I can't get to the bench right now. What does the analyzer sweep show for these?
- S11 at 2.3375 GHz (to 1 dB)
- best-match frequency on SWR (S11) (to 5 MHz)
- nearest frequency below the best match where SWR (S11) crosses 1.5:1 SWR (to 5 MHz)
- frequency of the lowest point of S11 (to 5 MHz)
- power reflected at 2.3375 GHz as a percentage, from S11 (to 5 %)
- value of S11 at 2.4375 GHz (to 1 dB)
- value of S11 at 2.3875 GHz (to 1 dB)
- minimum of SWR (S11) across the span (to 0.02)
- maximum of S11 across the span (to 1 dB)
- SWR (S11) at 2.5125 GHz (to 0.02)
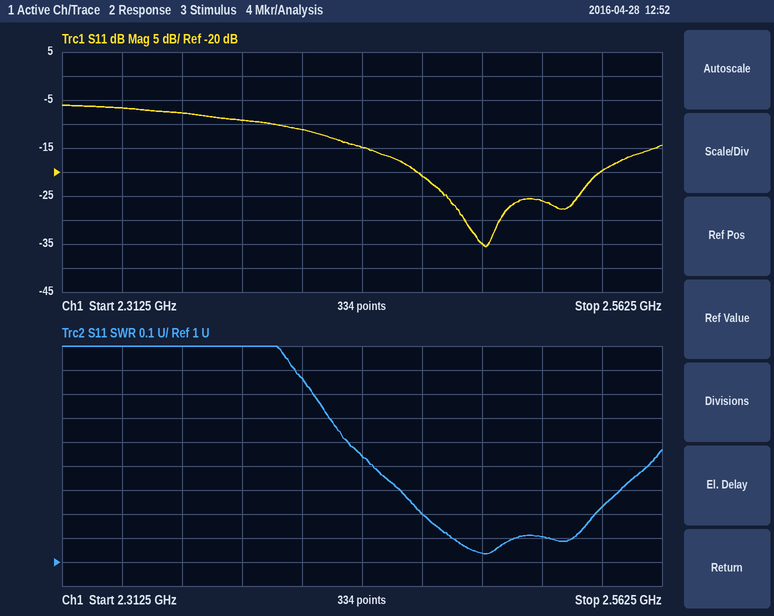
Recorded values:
-7 dB
2.490 GHz
2.430 GHz
2.490 GHz
20 %
-15 dB
-9 dB
1.04
-6 dB
1.10
